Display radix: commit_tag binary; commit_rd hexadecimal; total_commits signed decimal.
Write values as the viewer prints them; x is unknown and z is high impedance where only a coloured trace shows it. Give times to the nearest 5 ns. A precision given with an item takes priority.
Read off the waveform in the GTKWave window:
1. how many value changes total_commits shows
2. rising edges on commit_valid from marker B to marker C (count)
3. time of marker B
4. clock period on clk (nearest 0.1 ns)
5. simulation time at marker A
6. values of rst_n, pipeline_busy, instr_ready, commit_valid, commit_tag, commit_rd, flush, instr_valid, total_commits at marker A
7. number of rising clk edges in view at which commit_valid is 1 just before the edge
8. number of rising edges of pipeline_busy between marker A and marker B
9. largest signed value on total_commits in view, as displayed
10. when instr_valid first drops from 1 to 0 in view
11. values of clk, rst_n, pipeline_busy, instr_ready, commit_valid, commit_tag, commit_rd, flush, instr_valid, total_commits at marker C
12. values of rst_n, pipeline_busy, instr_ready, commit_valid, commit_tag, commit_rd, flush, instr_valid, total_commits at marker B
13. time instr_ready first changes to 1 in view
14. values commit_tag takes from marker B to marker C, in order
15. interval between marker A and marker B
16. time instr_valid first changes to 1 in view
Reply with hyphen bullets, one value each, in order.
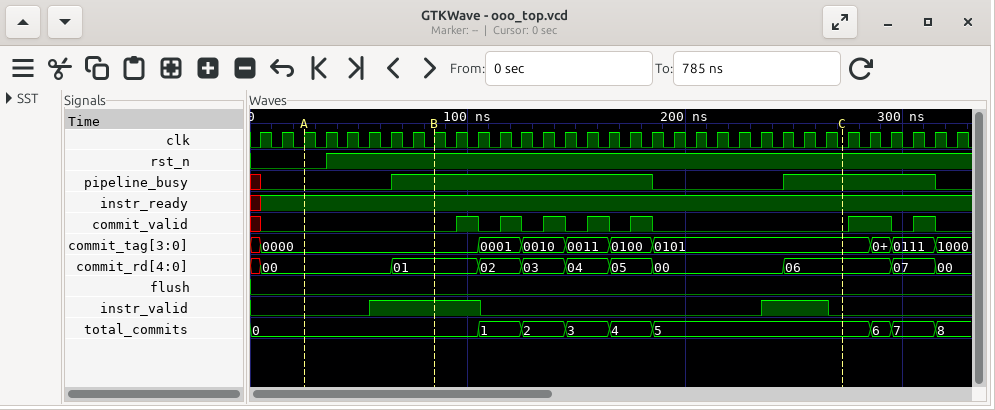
- 8
- 5
- 85 ns
- 10 ns
- 25 ns
- rst_n=0, pipeline_busy=0, instr_ready=1, commit_valid=0, commit_tag=0000, commit_rd=00, flush=0, instr_valid=0, total_commits=0
- 8
- 1
- 8
- 105 ns
- clk=0, rst_n=1, pipeline_busy=1, instr_ready=1, commit_valid=0, commit_tag=0101, commit_rd=06, flush=0, instr_valid=0, total_commits=5
- rst_n=1, pipeline_busy=1, instr_ready=1, commit_valid=0, commit_tag=0000, commit_rd=01, flush=0, instr_valid=1, total_commits=0
- 5 ns
- 0000, 0001, 0010, 0011, 0100, 0101
- 60 ns
- 55 ns
